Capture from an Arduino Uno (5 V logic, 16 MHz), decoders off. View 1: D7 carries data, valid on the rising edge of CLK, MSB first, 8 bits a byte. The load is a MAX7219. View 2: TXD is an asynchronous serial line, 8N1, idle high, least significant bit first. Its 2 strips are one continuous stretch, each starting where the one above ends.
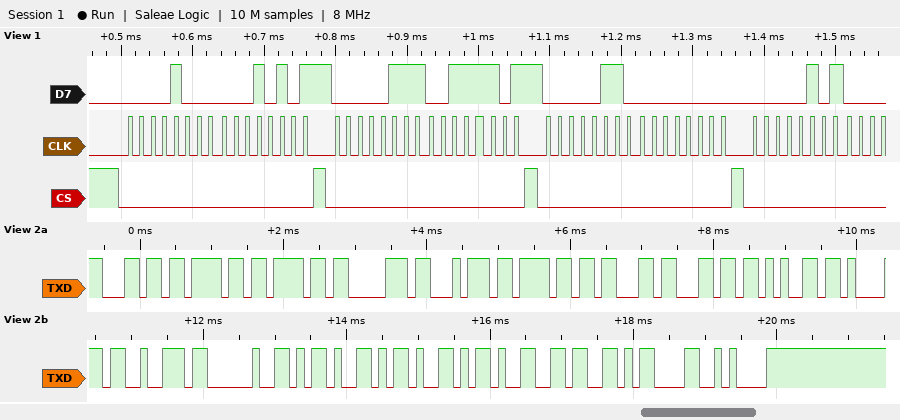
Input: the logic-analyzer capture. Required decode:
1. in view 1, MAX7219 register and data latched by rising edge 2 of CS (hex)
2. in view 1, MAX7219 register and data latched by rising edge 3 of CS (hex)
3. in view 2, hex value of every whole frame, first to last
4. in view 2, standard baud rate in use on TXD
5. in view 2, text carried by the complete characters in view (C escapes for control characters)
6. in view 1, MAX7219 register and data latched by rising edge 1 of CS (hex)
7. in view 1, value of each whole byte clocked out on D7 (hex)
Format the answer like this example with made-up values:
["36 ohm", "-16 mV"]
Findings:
["register 0x7, data 0x3D", "register 0x6, data 0x00", "0x6C 0x6F 0x6F 0x70 0x74 0x6F 0x63 0x6C 0x65 0x61 0x72 0x20 0x2D 0x2D 0x2D 0x36 0x0D 0x0A", "9600 baud", "\"looptoclear ---6\\r\\n\"", "register 0x8, data 0x15", "08 15 07 3D 06 00 05"]
